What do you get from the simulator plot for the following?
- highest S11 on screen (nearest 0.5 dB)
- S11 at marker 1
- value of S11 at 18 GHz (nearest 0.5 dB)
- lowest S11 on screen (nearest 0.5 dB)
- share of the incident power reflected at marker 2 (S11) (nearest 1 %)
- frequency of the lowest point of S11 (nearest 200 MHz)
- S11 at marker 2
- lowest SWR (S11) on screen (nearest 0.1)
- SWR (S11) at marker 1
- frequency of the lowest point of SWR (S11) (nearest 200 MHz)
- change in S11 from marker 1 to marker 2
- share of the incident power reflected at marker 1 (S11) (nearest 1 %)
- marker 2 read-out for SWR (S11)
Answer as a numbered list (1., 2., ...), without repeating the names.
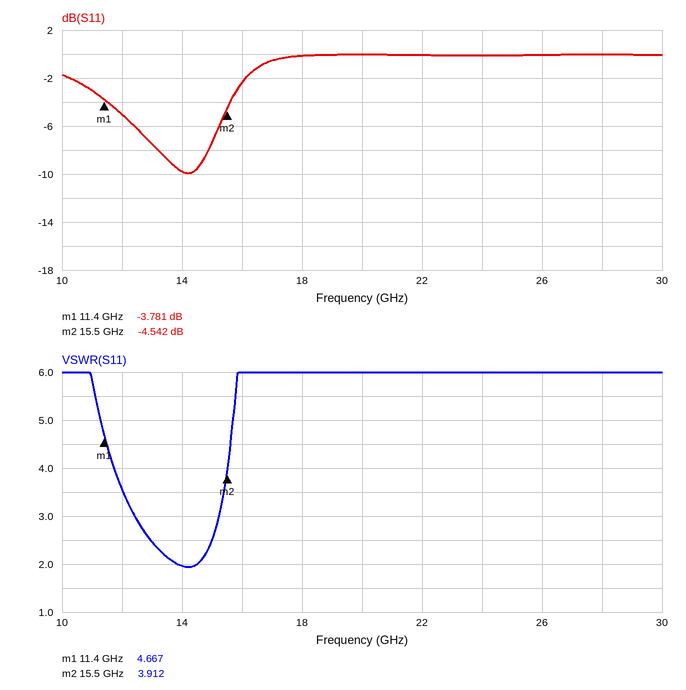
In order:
1. 0.0 dB
2. -3.781 dB
3. 0.0 dB
4. -10.0 dB
5. 35 %
6. 14.2 GHz
7. -4.542 dB
8. 1.9
9. 4.667
10. 14.2 GHz
11. -0.761 dB
12. 42 %
13. 3.912
